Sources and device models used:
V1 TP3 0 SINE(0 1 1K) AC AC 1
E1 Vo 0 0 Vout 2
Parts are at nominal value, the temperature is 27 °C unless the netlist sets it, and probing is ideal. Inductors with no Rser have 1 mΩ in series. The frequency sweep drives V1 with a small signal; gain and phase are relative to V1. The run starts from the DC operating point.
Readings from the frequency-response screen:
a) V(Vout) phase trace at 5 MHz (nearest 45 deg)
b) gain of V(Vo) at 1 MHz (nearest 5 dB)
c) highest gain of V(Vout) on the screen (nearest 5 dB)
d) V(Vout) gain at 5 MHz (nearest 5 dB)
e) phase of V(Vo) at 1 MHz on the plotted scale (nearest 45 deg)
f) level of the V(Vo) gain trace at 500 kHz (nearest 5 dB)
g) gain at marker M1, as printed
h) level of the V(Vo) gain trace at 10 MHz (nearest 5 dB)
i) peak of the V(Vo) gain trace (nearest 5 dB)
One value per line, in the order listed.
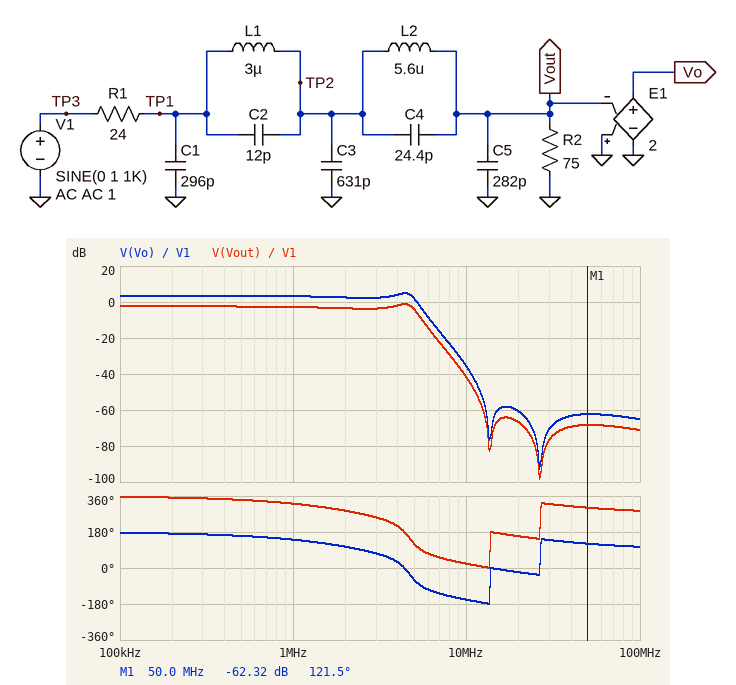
135 deg
5 dB
0 dB
-5 dB
135 deg
5 dB
-62.32 dB
-35 dB
5 dB
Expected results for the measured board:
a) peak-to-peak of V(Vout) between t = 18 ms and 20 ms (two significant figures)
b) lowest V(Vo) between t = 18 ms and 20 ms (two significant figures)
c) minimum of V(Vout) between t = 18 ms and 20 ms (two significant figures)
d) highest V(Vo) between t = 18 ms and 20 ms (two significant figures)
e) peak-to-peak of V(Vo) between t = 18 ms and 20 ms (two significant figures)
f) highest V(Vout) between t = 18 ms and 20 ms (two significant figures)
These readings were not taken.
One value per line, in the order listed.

1.5 V
-1.5 V
-760 mV
1.5 V
3.0 V
760 mV
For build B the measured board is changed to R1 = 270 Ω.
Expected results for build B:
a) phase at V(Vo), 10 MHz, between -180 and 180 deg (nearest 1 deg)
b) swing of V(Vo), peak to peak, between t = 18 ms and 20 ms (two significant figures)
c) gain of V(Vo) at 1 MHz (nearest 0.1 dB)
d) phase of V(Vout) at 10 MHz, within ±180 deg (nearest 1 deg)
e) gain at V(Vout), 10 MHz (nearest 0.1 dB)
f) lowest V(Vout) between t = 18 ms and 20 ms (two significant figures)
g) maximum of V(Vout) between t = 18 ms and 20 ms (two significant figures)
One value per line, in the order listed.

145 deg
870 mV
-6.9 dB
-35 deg
-53.1 dB
-220 mV
220 mV
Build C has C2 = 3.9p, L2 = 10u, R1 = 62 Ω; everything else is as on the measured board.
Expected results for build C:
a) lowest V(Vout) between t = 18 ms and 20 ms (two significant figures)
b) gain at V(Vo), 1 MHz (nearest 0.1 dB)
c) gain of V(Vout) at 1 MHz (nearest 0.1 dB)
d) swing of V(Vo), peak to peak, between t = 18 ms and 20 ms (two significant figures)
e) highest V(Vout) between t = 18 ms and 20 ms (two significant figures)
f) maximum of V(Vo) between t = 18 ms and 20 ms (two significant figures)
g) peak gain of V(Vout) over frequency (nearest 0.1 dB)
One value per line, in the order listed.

-550 mV
0.3 dB
-5.8 dB
2.2 V
550 mV
1.1 V
-5.2 dB
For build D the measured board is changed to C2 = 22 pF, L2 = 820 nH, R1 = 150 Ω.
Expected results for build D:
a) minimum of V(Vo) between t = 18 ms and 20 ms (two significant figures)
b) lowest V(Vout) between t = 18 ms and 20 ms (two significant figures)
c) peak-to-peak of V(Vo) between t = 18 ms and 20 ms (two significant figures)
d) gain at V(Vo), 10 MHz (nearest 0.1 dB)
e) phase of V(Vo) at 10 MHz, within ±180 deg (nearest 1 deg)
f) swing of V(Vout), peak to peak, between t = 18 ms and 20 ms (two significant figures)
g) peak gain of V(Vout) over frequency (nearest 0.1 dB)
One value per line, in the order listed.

-670 mV
-330 mV
1.3 V
-16.7 dB
-100 deg
670 mV
-9.5 dB
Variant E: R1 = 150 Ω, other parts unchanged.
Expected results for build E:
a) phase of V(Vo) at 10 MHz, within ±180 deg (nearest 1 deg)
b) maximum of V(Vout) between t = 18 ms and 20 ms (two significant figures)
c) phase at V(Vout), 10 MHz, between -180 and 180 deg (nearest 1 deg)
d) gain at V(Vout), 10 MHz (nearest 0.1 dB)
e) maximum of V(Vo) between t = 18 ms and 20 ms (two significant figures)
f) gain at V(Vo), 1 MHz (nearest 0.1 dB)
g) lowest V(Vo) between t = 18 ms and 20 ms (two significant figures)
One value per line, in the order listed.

156 deg
330 mV
-24 deg
-48.6 dB
670 mV
-3.3 dB
-670 mV
